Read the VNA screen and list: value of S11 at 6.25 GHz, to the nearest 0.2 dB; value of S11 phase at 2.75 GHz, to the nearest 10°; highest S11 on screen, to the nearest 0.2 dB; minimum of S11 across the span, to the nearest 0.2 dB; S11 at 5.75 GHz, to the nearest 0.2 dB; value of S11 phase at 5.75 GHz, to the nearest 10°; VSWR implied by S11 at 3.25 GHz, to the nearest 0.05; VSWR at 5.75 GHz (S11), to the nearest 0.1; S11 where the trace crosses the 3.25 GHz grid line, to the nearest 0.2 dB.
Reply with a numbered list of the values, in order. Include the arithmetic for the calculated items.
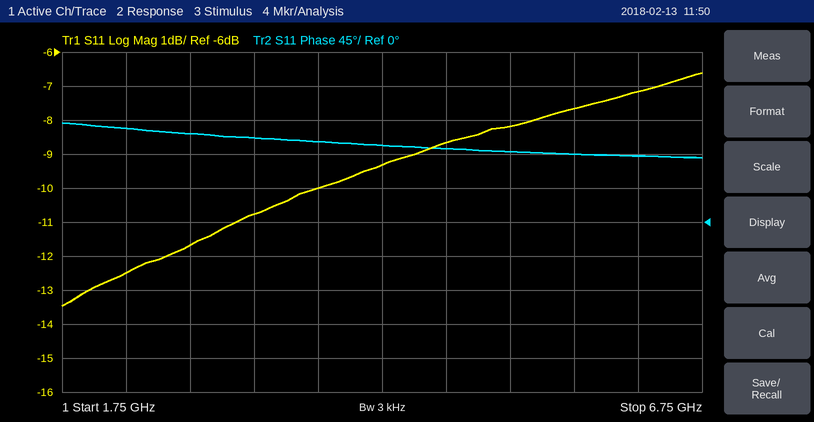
1. -7.2 dB
2. 120°
3. -6.6 dB
4. -13.4 dB
5. -7.6 dB
6. 90°
7. |Γ| = 10^(-10.8/20) = 0.2884; VSWR = (1 + 0.2884)/(1 − 0.2884) ≈ 1.81, so 1.80 to the nearest 0.05
8. |Γ| = 10^(-7.6/20) = 0.4169; VSWR = (1 + 0.4169)/(1 − 0.4169) ≈ 2.4
9. -10.8 dB
